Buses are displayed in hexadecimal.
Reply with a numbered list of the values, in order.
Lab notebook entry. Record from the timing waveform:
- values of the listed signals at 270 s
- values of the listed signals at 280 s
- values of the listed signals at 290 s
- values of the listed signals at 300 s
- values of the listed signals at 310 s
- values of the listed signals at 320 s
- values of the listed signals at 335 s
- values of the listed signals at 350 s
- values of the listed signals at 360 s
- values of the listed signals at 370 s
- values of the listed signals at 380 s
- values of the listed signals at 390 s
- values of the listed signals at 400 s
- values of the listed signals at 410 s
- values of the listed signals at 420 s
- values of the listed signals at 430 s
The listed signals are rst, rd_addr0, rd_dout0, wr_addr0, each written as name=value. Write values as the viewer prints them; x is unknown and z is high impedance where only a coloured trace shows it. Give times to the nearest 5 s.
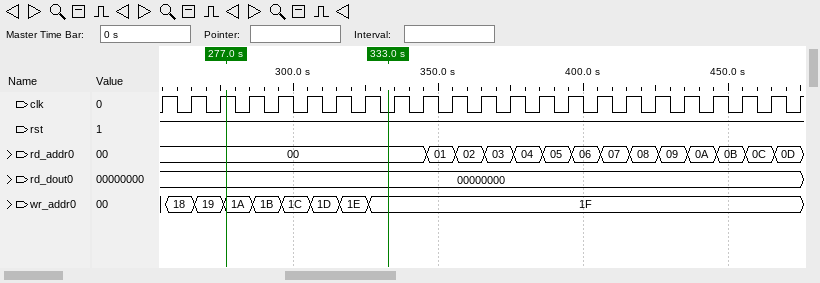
1. rst=1, rd_addr0=00, rd_dout0=00000000, wr_addr0=19
2. rst=1, rd_addr0=00, rd_dout0=00000000, wr_addr0=1A
3. rst=1, rd_addr0=00, rd_dout0=00000000, wr_addr0=1B
4. rst=1, rd_addr0=00, rd_dout0=00000000, wr_addr0=1C
5. rst=1, rd_addr0=00, rd_dout0=00000000, wr_addr0=1D
6. rst=1, rd_addr0=00, rd_dout0=00000000, wr_addr0=1E
7. rst=1, rd_addr0=00, rd_dout0=00000000, wr_addr0=1F
8. rst=1, rd_addr0=01, rd_dout0=00000000, wr_addr0=1F
9. rst=1, rd_addr0=02, rd_dout0=00000000, wr_addr0=1F
10. rst=1, rd_addr0=03, rd_dout0=00000000, wr_addr0=1F
11. rst=1, rd_addr0=04, rd_dout0=00000000, wr_addr0=1F
12. rst=1, rd_addr0=05, rd_dout0=00000000, wr_addr0=1F
13. rst=1, rd_addr0=06, rd_dout0=00000000, wr_addr0=1F
14. rst=1, rd_addr0=07, rd_dout0=00000000, wr_addr0=1F
15. rst=1, rd_addr0=08, rd_dout0=00000000, wr_addr0=1F
16. rst=1, rd_addr0=09, rd_dout0=00000000, wr_addr0=1F
